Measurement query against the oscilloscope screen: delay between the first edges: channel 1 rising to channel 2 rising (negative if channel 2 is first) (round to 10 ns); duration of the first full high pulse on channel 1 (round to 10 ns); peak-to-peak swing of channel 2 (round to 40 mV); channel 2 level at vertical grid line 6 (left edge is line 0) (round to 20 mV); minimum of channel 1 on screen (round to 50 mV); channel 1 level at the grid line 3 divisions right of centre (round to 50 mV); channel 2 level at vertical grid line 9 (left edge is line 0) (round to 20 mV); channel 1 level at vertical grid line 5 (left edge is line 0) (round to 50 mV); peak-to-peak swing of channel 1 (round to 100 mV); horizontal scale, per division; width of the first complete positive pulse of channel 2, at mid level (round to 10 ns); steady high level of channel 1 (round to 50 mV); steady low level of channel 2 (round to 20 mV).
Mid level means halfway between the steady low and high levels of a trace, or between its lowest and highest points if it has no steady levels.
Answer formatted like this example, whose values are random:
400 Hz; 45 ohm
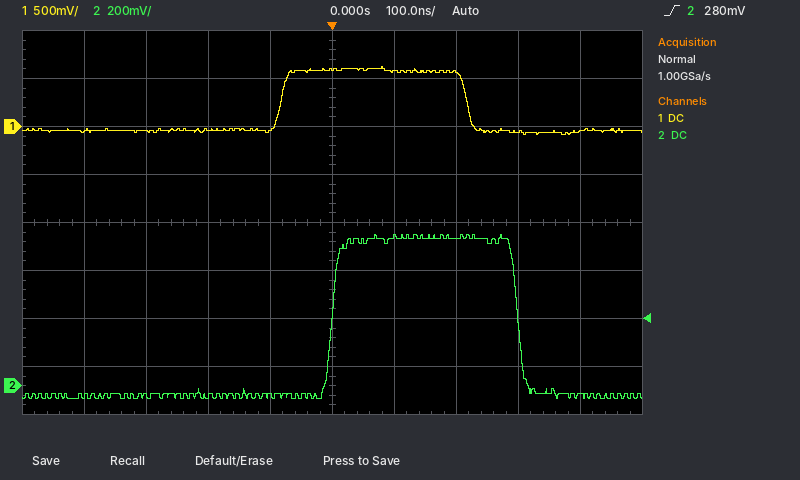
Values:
+80 ns; 300 ns; 680 mV; 620 mV; -100 mV; -50 mV; -40 mV; 600 mV; 700 mV; 100 ns; 300 ns; 600 mV; -40 mV
